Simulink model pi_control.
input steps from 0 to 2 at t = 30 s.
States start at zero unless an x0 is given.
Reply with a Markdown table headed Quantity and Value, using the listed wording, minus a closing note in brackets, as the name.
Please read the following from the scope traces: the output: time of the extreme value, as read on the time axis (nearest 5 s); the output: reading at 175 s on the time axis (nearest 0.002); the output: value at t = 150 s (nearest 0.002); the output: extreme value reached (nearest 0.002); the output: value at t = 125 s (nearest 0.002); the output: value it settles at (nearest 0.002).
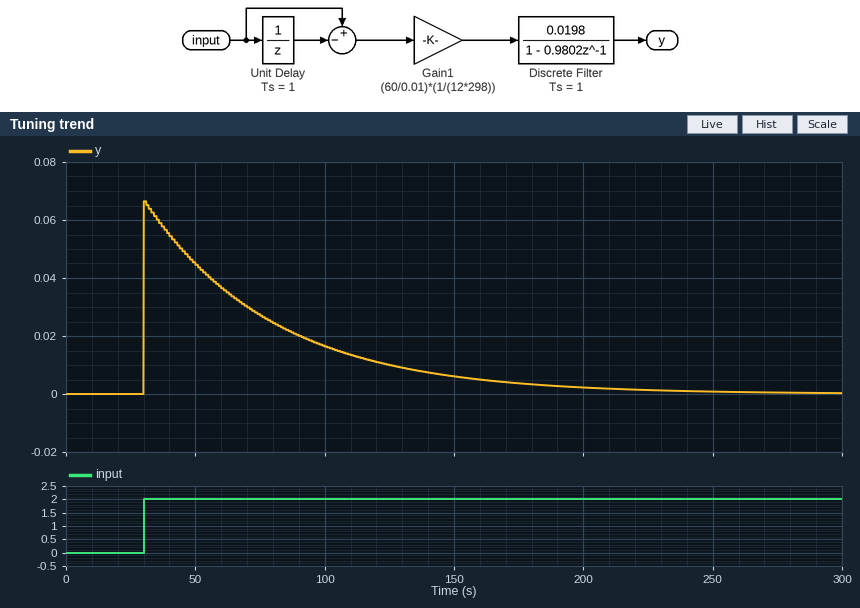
| Quantity | Value |
|---|---|
| the output: time of the extreme value, as read on the time axis | 30 s |
| the output: reading at 175 s on the time axis | 0.004 |
| the output: value at t = 150 s | 0.006 |
| the output: extreme value reached | 0.066 |
| the output: value at t = 125 s | 0.010 |
| the output: value it settles at | 0.000 |
